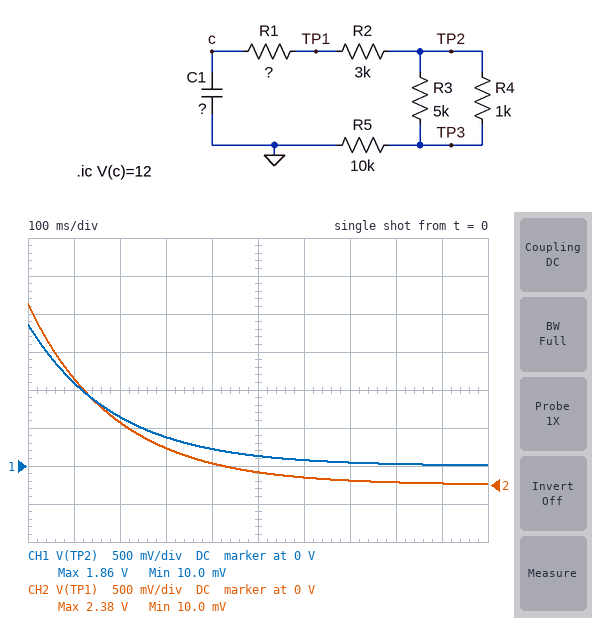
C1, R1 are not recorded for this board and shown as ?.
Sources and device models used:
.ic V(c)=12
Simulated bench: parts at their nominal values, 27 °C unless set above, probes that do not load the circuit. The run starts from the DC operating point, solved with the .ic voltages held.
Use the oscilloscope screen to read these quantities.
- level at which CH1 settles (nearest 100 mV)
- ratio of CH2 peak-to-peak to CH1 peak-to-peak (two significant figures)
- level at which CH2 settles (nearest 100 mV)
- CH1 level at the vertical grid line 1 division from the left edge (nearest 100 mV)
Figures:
0 V
1.3
0 V
1.1 V
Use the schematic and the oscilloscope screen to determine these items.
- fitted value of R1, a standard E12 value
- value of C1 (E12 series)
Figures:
56 kΩ
2.7 µF
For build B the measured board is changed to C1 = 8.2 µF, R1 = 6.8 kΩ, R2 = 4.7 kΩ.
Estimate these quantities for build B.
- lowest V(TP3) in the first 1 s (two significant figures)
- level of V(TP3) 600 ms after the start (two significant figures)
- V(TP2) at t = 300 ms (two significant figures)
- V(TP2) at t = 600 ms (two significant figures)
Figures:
23 mV
200 mV
1.1 V
220 mV
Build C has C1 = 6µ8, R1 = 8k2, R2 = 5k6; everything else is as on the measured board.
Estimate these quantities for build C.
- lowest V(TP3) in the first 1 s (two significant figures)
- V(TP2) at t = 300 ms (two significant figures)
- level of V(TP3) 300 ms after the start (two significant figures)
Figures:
12 mV
880 mV
810 mV
